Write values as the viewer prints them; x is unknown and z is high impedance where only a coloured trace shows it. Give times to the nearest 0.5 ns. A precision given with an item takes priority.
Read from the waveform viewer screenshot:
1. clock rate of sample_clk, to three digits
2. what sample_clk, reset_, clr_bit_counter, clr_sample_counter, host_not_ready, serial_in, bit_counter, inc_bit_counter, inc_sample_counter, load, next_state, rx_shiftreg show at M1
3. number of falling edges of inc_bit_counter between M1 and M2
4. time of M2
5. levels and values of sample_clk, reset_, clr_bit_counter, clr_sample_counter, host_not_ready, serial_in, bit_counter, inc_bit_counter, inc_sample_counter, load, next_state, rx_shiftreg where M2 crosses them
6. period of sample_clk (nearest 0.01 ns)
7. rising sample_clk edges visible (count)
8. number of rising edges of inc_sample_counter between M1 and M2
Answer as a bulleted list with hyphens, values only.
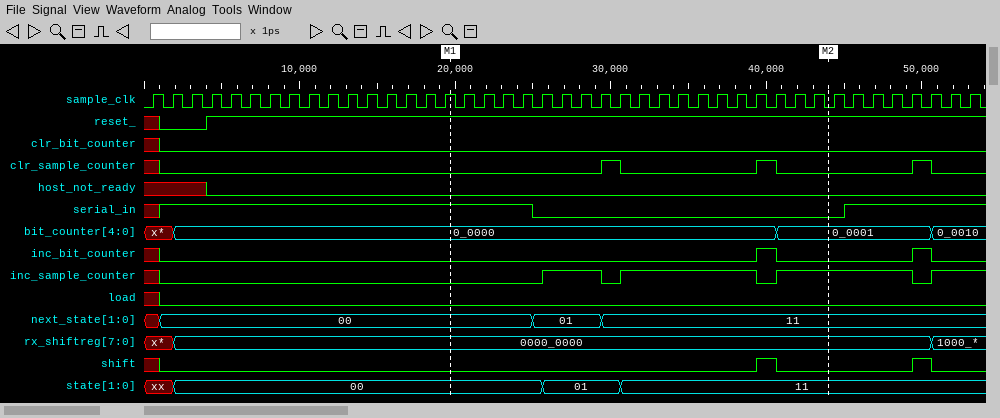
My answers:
- 800 MHz
- sample_clk=1, reset_=1, clr_bit_counter=0, clr_sample_counter=0, host_not_ready=0, serial_in=1, bit_counter=0_0000, inc_bit_counter=0, inc_sample_counter=0, load=0, next_state=00, rx_shiftreg=0000_0000
- 1
- 44 ns
- sample_clk=0, reset_=1, clr_bit_counter=0, clr_sample_counter=0, host_not_ready=0, serial_in=0, bit_counter=0_0001, inc_bit_counter=0, inc_sample_counter=1, load=0, next_state=11, rx_shiftreg=0000_0000
- 1.25 ns
- 43
- 3
